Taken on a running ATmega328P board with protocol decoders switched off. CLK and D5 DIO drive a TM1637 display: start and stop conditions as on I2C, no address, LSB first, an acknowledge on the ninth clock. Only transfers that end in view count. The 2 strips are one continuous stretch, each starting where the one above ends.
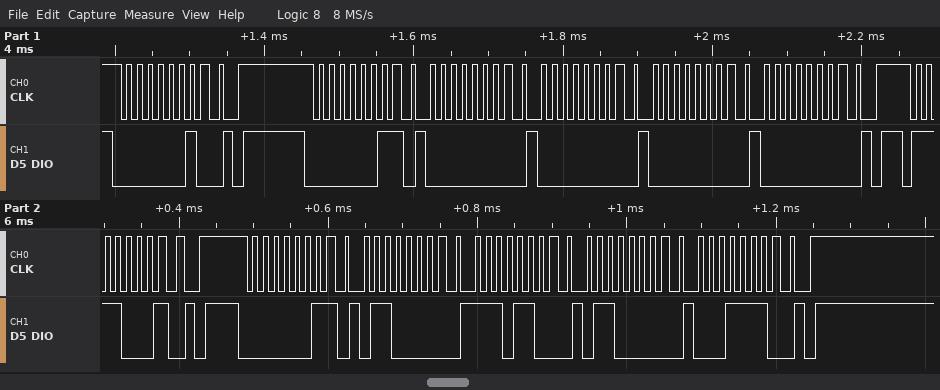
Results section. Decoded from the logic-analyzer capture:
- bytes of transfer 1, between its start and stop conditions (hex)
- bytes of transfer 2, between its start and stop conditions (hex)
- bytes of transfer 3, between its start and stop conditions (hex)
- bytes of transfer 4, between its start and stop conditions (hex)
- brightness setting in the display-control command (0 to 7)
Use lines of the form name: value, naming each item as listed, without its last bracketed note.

bytes of transfer 1, between its start and stop conditions: 40
bytes of transfer 2, between its start and stop conditions: C0 00 00 00 00
bytes of transfer 3, between its start and stop conditions: 8F
bytes of transfer 4, between its start and stop conditions: C0 06 37 06 78
brightness setting in the display-control command: 7
